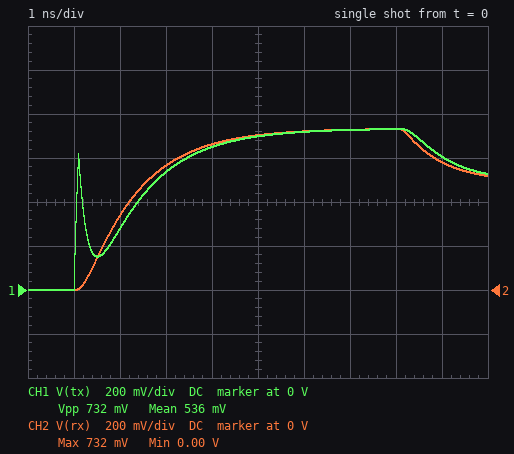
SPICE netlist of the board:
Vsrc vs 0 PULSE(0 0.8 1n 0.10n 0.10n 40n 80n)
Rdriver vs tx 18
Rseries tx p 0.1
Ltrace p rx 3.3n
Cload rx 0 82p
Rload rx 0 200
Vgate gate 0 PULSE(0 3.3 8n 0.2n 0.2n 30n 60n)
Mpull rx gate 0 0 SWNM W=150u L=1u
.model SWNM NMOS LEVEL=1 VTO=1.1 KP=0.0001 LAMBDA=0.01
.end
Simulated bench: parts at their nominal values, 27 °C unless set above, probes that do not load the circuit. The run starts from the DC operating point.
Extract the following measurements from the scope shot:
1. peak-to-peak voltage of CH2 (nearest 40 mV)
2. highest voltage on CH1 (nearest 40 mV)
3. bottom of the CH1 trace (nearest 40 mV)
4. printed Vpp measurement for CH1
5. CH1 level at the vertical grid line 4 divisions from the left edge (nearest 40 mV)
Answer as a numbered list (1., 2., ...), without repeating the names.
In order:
1. 720 mV
2. 720 mV
3. 0 V
4. 732 mV
5. 640 mV
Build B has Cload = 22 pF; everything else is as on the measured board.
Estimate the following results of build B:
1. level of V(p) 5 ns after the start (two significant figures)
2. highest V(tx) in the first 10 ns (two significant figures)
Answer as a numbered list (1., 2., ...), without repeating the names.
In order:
1. 730 mV
2. 750 mV
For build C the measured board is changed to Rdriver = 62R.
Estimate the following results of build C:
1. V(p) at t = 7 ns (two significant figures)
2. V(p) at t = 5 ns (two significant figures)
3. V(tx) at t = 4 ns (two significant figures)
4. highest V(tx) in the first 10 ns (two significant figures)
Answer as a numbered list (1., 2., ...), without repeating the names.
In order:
1. 480 mV
2. 390 mV
3. 320 mV
4. 510 mV
